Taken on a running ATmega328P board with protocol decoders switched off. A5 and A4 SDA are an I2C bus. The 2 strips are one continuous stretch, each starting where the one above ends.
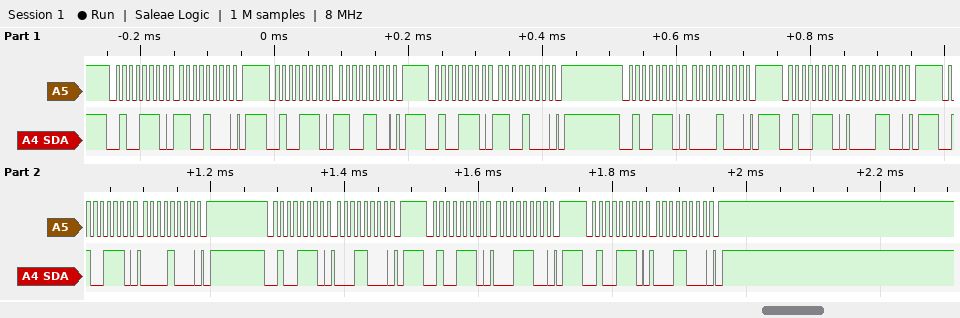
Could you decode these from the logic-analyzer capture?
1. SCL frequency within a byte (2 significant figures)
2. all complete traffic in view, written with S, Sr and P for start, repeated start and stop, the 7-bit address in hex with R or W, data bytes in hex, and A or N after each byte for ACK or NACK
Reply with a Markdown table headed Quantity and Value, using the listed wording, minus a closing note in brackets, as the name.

| Quantity | Value |
|---|---|
| SCL frequency within a byte | 100 kHz |
| all complete traffic in view, written with S, Sr and P for start, repeated start and stop, the 7-bit address in hex with R or W, data bytes in hex, and A or N after each byte for ACK or NACK | S 27W A C8 A P S 27W A CC A P S 27W A C8 A P S 27W A 08 A P S 27W A 0C A P S 27W A 08 A P S 27W A 18 A P S 27W A 1C A P S 27W A 18 A P |
